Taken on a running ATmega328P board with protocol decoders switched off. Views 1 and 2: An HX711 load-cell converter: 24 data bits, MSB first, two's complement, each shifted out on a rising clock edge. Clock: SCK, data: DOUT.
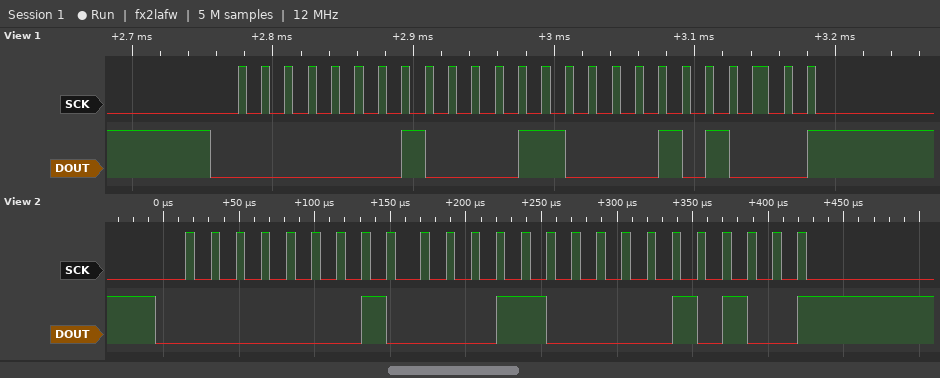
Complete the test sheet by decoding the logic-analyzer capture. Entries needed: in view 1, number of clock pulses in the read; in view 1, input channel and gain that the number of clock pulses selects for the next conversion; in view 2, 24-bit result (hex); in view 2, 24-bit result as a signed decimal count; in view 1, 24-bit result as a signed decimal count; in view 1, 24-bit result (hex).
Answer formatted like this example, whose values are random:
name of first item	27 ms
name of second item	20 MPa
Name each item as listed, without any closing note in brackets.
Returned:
in view 1, number of clock pulses in the read	25
in view 1, input channel and gain that the number of clock pulses selects for the next conversion	channel A, gain 128
in view 2, 24-bit result	0x010C14
in view 2, 24-bit result as a signed decimal count	68628
in view 1, 24-bit result as a signed decimal count	68648
in view 1, 24-bit result	0x010C28
